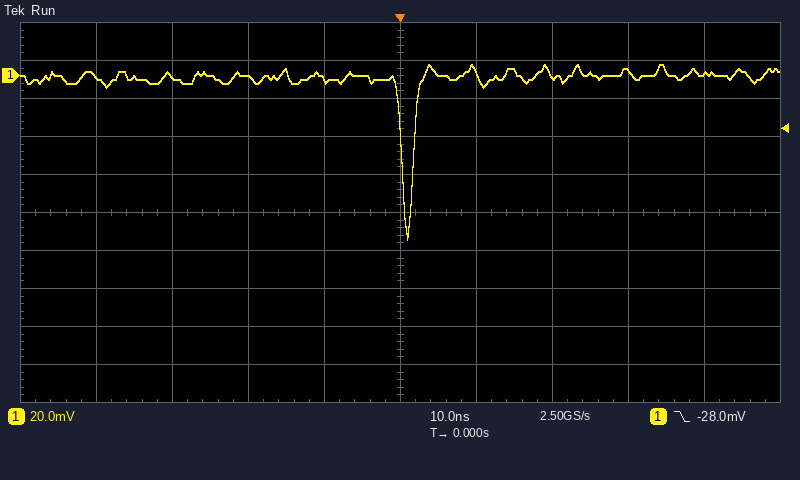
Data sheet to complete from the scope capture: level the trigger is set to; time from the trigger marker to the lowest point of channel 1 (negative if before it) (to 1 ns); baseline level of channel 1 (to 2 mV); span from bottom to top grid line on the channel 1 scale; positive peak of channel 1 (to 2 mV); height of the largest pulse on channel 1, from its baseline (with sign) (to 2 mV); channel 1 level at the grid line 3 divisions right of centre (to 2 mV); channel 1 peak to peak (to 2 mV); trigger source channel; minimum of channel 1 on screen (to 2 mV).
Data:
-28.0 mV
+1 ns
0 mV
200 mV
6 mV
-86 mV
2 mV
92 mV
channel 1
-86 mV
